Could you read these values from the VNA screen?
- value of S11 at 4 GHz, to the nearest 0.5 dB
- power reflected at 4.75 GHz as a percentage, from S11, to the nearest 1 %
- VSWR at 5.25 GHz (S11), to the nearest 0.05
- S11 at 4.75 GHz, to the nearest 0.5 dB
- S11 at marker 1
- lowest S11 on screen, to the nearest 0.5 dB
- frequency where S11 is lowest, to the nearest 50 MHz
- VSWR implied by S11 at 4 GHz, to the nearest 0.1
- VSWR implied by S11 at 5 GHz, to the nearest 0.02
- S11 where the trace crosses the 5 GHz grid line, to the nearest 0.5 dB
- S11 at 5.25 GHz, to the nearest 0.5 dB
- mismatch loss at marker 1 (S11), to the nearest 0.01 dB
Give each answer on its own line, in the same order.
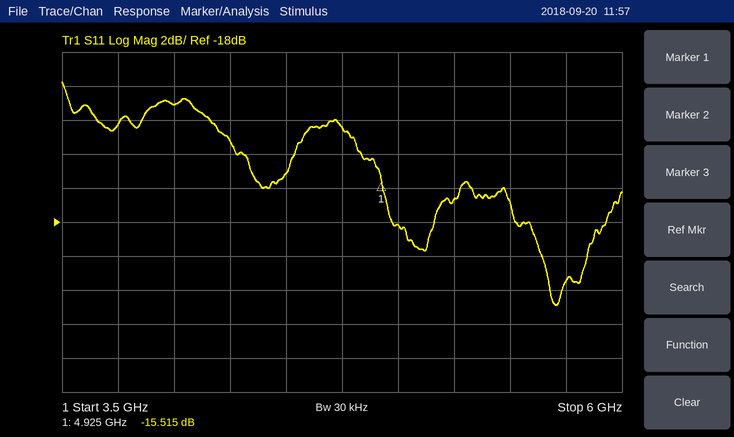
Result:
-11.0 dB
6 %
1.35
-12.5 dB
-15.515 dB
-23.0 dB
5.70 GHz
1.8
1.28
-18.0 dB
-16.5 dB
0.12 dB
